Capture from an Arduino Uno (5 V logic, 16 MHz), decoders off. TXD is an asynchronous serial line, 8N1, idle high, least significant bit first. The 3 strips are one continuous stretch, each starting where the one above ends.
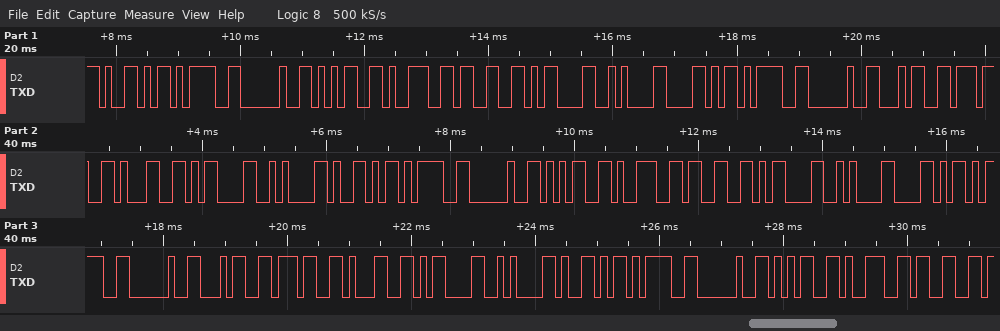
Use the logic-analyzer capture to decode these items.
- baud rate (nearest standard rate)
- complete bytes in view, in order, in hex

9600 baud
59 3D 20 35 39 33 0D 0A 58 3D 20 34 37 31 0D 0A 59 3D 20 35 39 33 0D 0A 58 3D 20 34 37 31 0D 0A 59 3D 20 35 39 33
